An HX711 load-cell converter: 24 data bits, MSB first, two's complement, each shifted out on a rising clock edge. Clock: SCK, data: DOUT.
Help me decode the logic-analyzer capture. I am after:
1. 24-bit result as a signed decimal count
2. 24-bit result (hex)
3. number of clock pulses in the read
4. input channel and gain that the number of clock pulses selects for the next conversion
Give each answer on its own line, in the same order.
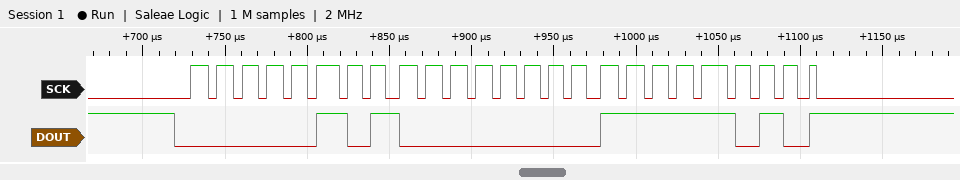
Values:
327930
0x0500FA
25
channel A, gain 128
